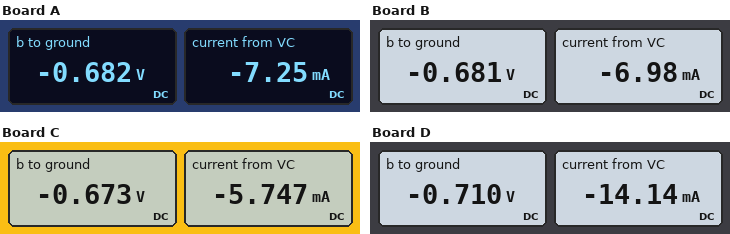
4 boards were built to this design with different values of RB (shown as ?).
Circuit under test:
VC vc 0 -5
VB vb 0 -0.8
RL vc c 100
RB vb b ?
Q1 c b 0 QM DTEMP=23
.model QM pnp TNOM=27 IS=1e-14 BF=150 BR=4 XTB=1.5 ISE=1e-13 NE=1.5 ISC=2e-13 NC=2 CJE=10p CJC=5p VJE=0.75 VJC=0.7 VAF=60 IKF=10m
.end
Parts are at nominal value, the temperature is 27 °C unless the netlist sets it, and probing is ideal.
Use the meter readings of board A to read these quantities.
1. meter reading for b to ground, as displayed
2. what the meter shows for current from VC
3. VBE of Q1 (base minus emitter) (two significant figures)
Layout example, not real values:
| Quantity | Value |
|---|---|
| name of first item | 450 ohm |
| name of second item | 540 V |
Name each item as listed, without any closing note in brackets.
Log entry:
| Quantity | Value |
|---|---|
| meter reading for b to ground, as displayed | -0.682 V |
| what the meter shows for current from VC | -7.25 mA |
| VBE of Q1 (base minus emitter) | -680 mV |
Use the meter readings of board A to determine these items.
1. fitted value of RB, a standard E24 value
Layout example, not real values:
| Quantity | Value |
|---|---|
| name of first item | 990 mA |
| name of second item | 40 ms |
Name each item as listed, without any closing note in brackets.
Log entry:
| Quantity | Value |
|---|---|
| fitted value of RB, a standard E24 value | 1.5 kΩ |
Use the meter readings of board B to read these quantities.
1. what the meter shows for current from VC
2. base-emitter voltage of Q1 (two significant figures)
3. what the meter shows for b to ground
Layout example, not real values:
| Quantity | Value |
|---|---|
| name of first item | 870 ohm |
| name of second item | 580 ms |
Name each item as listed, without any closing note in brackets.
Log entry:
| Quantity | Value |
|---|---|
| what the meter shows for current from VC | -6.98 mA |
| base-emitter voltage of Q1 | -680 mV |
| what the meter shows for b to ground | -0.681 V |
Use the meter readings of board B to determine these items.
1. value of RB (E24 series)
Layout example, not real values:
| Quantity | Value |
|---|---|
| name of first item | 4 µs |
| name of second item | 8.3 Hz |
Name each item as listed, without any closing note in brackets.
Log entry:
| Quantity | Value |
|---|---|
| value of RB | 1.6 kΩ |
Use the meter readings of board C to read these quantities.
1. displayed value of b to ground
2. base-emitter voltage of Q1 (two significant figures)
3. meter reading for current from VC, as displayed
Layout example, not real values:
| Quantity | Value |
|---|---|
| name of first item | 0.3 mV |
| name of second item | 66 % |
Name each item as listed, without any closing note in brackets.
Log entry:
| Quantity | Value |
|---|---|
| displayed value of b to ground | -0.673 V |
| base-emitter voltage of Q1 | -670 mV |
| meter reading for current from VC, as displayed | -5.747 mA |
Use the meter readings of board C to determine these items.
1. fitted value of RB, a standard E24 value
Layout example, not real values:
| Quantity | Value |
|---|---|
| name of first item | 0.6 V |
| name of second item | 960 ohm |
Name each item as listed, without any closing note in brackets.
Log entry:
| Quantity | Value |
|---|---|
| fitted value of RB, a standard E24 value | 2.2 kΩ |
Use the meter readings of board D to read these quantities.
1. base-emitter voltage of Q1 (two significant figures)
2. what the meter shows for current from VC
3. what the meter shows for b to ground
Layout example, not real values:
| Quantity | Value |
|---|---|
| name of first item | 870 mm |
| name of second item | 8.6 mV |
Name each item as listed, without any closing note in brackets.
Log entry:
| Quantity | Value |
|---|---|
| base-emitter voltage of Q1 | -710 mV |
| what the meter shows for current from VC | -14.14 mA |
| what the meter shows for b to ground | -0.710 V |
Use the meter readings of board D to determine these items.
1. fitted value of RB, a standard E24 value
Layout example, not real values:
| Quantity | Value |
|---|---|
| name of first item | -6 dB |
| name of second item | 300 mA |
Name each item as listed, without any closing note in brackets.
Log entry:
| Quantity | Value |
|---|---|
| fitted value of RB, a standard E24 value | 430 Ω |
